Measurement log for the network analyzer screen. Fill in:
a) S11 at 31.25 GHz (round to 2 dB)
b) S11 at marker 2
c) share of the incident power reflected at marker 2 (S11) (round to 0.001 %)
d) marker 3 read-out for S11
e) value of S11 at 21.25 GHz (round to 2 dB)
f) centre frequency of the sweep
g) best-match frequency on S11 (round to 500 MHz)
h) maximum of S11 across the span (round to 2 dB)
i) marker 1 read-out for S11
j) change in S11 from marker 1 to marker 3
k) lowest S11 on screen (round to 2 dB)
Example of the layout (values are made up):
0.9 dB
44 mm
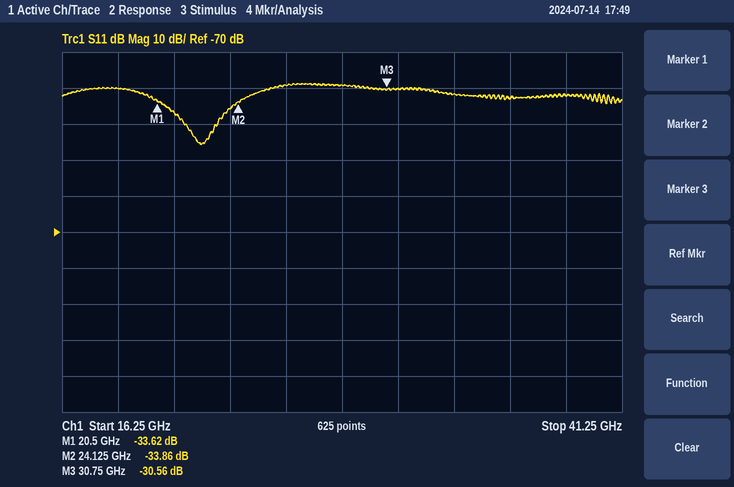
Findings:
-30 dB
-33.86 dB
0.041 %
-30.56 dB
-36 dB
28.75 GHz
22.5 GHz
-28 dB
-33.62 dB
3.06 dB
-46 dB
